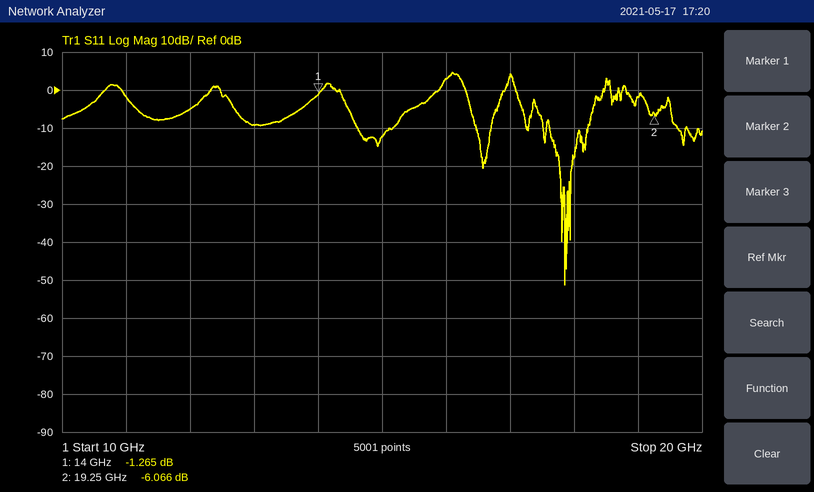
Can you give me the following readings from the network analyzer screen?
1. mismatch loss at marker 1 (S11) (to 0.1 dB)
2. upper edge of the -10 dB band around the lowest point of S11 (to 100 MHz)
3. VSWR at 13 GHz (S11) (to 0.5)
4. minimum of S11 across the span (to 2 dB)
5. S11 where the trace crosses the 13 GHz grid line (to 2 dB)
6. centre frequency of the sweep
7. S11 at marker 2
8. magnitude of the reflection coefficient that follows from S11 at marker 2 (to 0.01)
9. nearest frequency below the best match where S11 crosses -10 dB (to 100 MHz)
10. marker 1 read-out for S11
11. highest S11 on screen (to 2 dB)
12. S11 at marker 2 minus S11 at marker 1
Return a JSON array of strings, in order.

["6.0 dB", "18.2 GHz", "2.0", "-52 dB", "-10 dB", "15 GHz", "-6.066 dB", "0.50", "17.6 GHz", "-1.265 dB", "4 dB", "-4.801 dB"]
